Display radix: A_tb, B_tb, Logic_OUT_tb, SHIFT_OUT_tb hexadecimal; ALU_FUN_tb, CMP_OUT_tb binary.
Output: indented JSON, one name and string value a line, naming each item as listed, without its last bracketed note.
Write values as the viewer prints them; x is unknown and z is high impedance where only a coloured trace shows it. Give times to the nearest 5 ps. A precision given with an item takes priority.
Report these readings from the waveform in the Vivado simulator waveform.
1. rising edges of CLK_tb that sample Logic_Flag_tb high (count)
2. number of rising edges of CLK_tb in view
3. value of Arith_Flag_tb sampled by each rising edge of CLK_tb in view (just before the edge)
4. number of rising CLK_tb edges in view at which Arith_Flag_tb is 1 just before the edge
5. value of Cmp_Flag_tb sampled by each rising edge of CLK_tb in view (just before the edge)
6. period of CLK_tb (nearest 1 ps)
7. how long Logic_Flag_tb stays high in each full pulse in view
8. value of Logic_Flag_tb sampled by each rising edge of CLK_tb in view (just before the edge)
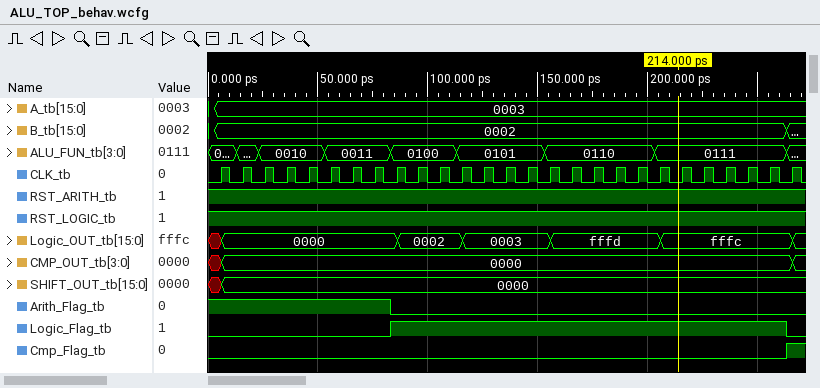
{
  "rising edges of CLK_tb that sample Logic_Flag_tb high": "18",
  "number of rising edges of CLK_tb in view": "27",
  "value of Arith_Flag_tb sampled by each rising edge of CLK_tb in view": "1 1 1 1 1 1 1 1 0 0 0 0 0 0 0 0 0 0 0 0 0 0 0 0 0 0 0",
  "number of rising CLK_tb edges in view at which Arith_Flag_tb is 1 just before the edge": "8",
  "value of Cmp_Flag_tb sampled by each rising edge of CLK_tb in view": "0 0 0 0 0 0 0 0 0 0 0 0 0 0 0 0 0 0 0 0 0 0 0 0 0 0 1",
  "period of CLK_tb": "10 ps",
  "how long Logic_Flag_tb stays high in each full pulse in view": "180 ps",
  "value of Logic_Flag_tb sampled by each rising edge of CLK_tb in view": "0 0 0 0 0 0 0 0 1 1 1 1 1 1 1 1 1 1 1 1 1 1 1 1 1 1 0"
}
